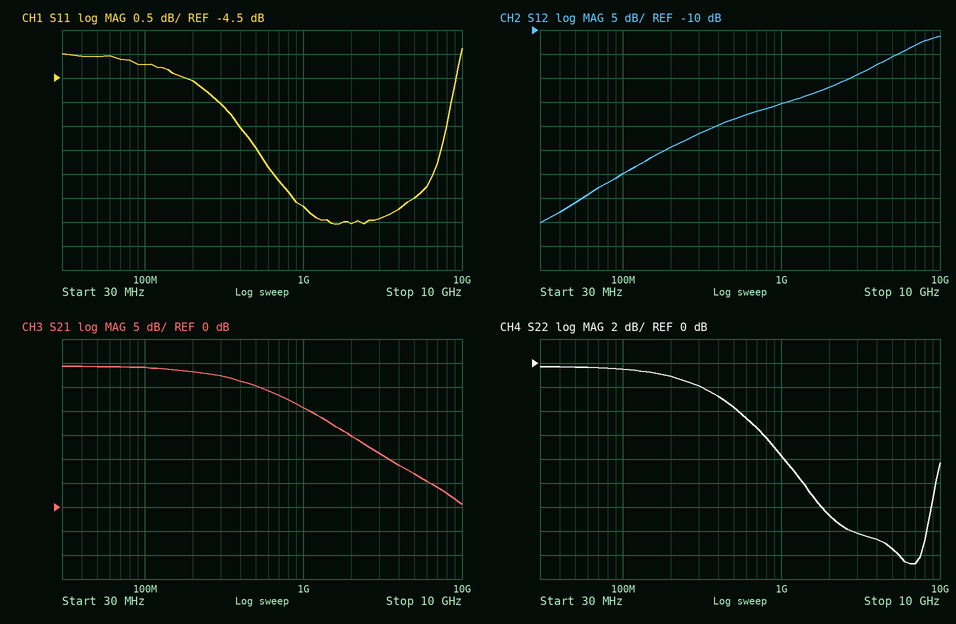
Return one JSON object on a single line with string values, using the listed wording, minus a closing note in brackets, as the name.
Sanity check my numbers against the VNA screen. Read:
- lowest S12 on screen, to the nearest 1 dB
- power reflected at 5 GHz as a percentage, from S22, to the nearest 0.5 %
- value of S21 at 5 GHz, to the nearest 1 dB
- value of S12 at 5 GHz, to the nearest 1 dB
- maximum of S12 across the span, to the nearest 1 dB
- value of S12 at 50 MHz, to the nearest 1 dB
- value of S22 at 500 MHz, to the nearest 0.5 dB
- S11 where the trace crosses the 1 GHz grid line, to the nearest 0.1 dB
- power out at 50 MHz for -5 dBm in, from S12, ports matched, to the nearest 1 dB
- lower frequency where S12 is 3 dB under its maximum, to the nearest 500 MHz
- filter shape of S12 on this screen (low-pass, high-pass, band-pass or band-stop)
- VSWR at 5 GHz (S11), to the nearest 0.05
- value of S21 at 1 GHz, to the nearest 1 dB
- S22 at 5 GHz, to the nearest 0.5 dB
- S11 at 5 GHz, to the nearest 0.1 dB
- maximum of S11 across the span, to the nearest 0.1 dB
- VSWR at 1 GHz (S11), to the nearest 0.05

{"lowest S12 on screen, to the nearest 1 dB": "-50 dB", "power reflected at 5 GHz as a percentage, from S22, to the nearest 0.5 %": "3.0 %", "value of S21 at 5 GHz, to the nearest 1 dB": "7 dB", "value of S12 at 5 GHz, to the nearest 1 dB": "-16 dB", "maximum of S12 across the span, to the nearest 1 dB": "-11 dB", "value of S12 at 50 MHz, to the nearest 1 dB": "-46 dB", "value of S22 at 500 MHz, to the nearest 0.5 dB": "-3.5 dB", "S11 where the trace crosses the 1 GHz grid line, to the nearest 0.1 dB": "-7.2 dB", "power out at 50 MHz for -5 dBm in, from S12, ports matched, to the nearest 1 dB": "-51 dBm", "lower frequency where S12 is 3 dB under its maximum, to the nearest 500 MHz": "6.0 GHz", "filter shape of S12 on this screen": "high-pass", "VSWR at 5 GHz (S11), to the nearest 0.05": "2.60", "value of S21 at 1 GHz, to the nearest 1 dB": "21 dB", "S22 at 5 GHz, to the nearest 0.5 dB": "-15.5 dB", "S11 at 5 GHz, to the nearest 0.1 dB": "-7.0 dB", "maximum of S11 across the span, to the nearest 0.1 dB": "-3.9 dB", "VSWR at 1 GHz (S11), to the nearest 0.05": "2.55"}
